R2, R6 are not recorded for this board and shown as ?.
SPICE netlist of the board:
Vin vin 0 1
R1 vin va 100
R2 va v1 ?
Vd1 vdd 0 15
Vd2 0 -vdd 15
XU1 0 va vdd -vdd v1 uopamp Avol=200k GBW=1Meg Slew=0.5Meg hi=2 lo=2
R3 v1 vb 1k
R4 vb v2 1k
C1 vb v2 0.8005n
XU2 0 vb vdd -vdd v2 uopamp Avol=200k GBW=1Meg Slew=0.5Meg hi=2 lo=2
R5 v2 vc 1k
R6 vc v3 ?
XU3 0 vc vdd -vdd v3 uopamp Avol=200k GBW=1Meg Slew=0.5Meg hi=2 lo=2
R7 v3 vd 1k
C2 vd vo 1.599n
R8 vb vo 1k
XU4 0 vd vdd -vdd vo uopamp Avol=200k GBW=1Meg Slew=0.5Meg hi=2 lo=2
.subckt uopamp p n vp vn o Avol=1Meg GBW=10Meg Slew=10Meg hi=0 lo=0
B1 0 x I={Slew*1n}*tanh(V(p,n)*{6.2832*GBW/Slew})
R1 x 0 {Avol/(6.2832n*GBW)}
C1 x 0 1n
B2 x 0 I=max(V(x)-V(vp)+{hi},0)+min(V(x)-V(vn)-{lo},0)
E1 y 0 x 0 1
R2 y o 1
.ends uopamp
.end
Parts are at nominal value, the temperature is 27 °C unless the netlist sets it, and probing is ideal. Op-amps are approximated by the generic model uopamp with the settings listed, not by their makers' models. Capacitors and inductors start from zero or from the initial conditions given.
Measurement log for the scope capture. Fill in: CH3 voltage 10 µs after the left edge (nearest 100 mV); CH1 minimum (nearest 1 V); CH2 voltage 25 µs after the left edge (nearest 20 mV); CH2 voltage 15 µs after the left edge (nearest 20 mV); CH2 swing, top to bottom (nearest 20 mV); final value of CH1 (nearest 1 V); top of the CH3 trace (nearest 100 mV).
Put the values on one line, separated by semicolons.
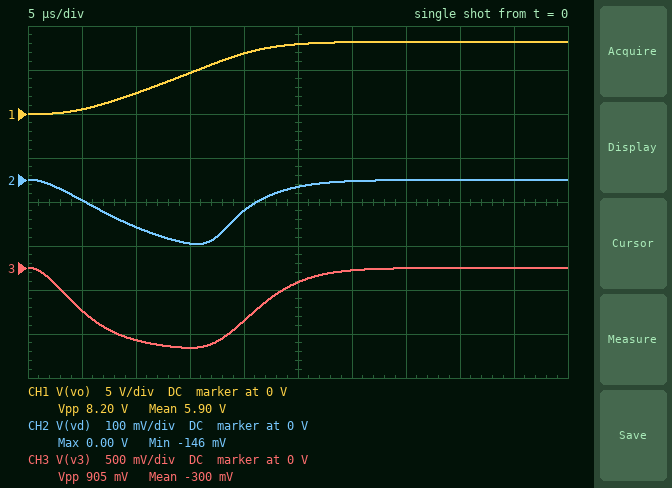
-800 mV; 0 V; -20 mV; -140 mV; 140 mV; 8 V; 0 V
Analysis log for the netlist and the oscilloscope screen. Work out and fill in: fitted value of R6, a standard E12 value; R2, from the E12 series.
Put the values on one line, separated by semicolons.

330 Ω; 820 Ω
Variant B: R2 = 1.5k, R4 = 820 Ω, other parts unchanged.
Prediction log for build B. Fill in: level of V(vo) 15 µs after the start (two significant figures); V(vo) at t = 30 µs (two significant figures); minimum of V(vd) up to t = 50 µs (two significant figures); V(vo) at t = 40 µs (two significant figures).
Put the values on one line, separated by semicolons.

4.3 V; 11 V; -160 mV; 13 V
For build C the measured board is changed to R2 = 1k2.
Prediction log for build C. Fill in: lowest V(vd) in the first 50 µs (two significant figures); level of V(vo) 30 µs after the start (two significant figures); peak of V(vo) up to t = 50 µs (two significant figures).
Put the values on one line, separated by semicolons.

-170 mV; 11 V; 12 V
